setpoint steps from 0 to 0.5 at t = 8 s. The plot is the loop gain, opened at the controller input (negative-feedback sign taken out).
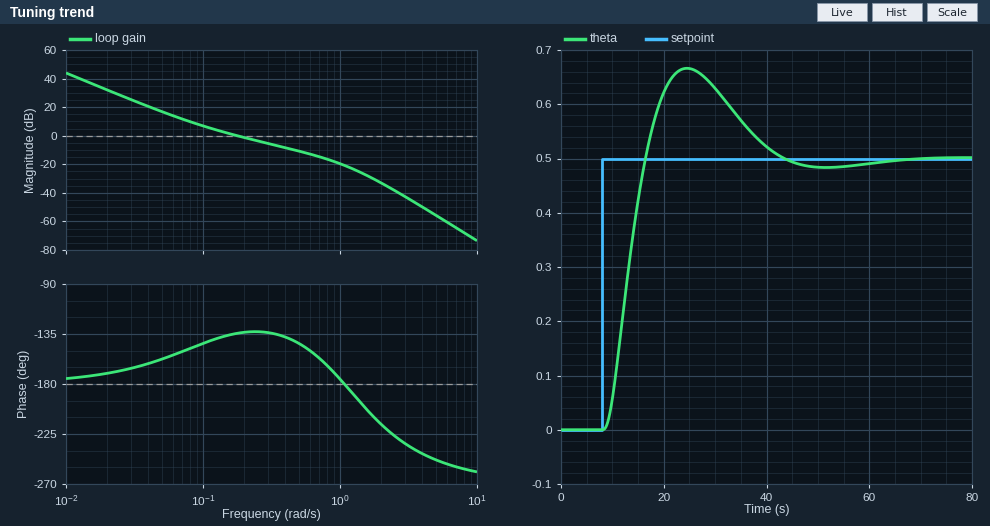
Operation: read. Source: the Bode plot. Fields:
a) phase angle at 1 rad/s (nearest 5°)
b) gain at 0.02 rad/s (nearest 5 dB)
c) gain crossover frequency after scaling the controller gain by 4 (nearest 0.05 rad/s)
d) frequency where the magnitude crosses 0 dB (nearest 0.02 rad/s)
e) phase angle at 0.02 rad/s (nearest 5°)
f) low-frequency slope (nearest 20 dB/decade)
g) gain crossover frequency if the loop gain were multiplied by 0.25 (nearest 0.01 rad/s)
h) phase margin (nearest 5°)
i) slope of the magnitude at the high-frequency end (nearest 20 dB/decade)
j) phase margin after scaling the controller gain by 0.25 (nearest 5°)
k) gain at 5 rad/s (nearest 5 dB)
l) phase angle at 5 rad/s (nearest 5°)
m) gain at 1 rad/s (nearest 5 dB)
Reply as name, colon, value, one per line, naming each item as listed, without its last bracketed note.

phase angle at 1 rad/s: -175°
gain at 0.02 rad/s: 30 dB
gain crossover frequency after scaling the controller gain by 4: 0.55 rad/s
frequency where the magnitude crosses 0 dB: 0.18 rad/s
phase angle at 0.02 rad/s: -170°
low-frequency slope: -40 dB/decade
gain crossover frequency if the loop gain were multiplied by 0.25: 0.07 rad/s
phase margin: 45°
slope of the magnitude at the high-frequency end: -60 dB/decade
phase margin after scaling the controller gain by 0.25: 30°
gain at 5 rad/s: -55 dB
phase angle at 5 rad/s: -250°
gain at 1 rad/s: -20 dB
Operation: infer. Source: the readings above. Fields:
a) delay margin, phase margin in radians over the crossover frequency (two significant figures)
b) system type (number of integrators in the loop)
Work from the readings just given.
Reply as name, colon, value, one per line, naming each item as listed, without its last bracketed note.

delay margin, phase margin in radians over the crossover frequency: 4.4 s
system type: 2
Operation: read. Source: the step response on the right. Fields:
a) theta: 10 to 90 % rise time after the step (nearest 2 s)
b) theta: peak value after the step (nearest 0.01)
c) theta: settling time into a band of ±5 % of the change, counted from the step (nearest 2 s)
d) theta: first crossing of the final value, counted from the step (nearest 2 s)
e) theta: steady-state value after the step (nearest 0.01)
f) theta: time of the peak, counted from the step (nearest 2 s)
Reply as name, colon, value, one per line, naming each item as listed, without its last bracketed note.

theta: 10 to 90 % rise time after the step: 6 s
theta: peak value after the step: 0.67
theta: settling time into a band of ±5 % of the change, counted from the step: 32 s
theta: first crossing of the final value, counted from the step: 8 s
theta: steady-state value after the step: 0.50
theta: time of the peak, counted from the step: 16 s
